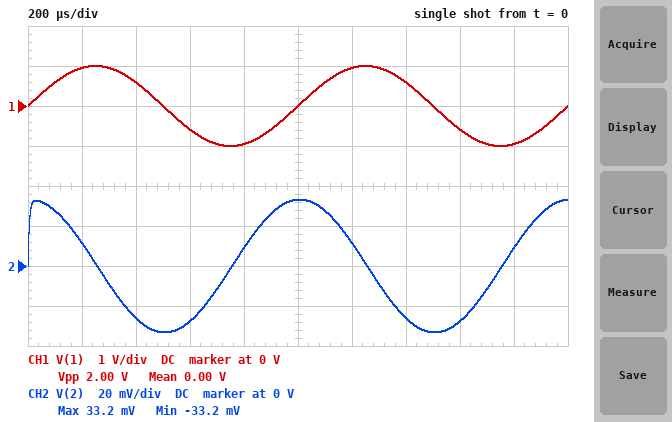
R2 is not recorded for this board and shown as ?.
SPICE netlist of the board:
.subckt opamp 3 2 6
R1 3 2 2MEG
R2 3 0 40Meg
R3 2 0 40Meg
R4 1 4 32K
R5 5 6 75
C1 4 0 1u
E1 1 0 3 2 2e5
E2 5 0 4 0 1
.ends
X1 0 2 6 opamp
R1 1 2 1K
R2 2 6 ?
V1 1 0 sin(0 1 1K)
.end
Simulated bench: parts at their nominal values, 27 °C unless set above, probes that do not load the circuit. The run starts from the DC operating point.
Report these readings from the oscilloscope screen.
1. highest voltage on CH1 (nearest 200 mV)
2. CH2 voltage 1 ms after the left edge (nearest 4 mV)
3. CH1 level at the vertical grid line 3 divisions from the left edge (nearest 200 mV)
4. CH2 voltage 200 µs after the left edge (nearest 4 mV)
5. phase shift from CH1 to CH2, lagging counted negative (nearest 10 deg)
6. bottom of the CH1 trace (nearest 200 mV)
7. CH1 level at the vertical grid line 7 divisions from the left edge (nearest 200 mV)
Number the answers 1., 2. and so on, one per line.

1. 1.0 V
2. 32 mV
3. -600 mV
4. 12 mV
5. 90 deg
6. -1.0 V
7. 600 mV
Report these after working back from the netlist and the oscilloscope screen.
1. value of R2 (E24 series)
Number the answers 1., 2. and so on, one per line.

1. 33 kΩ
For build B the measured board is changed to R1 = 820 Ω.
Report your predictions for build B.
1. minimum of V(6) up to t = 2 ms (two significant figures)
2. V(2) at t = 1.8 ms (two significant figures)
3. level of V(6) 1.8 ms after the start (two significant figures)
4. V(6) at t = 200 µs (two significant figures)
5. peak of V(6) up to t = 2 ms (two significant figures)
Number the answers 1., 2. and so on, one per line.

1. -40 V
2. 11 mV
3. 39 V
4. -38 V
5. 40 V
